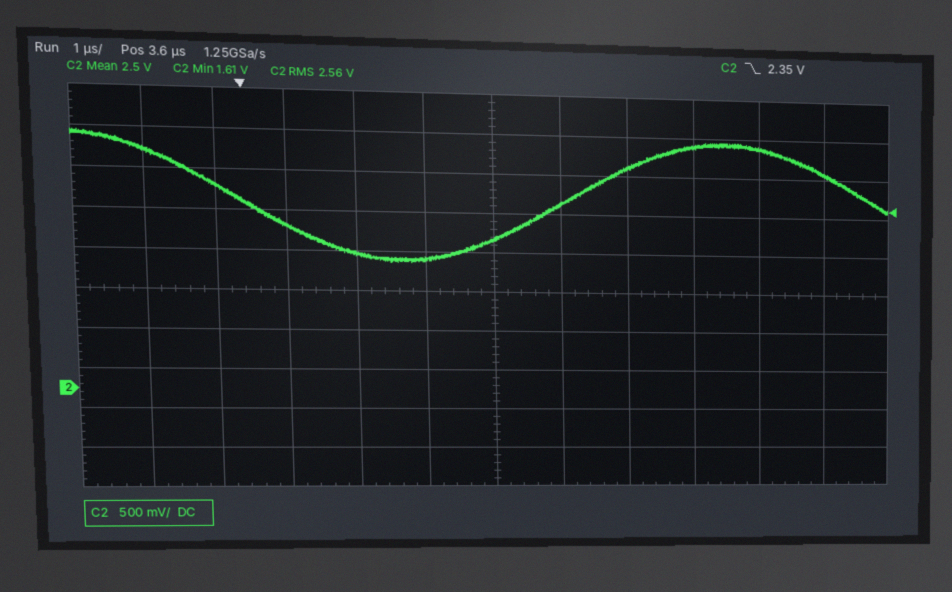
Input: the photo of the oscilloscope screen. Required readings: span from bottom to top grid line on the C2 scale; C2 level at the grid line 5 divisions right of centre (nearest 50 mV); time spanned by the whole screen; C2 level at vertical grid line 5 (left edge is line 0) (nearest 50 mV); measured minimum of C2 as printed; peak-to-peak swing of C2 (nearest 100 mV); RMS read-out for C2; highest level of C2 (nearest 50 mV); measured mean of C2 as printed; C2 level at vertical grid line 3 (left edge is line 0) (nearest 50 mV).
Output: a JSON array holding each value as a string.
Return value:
["5 V", "2.80 V", "12 µs", "1.65 V", "1.61 V", "1.60 V", "2.56 V", "3.20 V", "2.5 V", "2.05 V"]
